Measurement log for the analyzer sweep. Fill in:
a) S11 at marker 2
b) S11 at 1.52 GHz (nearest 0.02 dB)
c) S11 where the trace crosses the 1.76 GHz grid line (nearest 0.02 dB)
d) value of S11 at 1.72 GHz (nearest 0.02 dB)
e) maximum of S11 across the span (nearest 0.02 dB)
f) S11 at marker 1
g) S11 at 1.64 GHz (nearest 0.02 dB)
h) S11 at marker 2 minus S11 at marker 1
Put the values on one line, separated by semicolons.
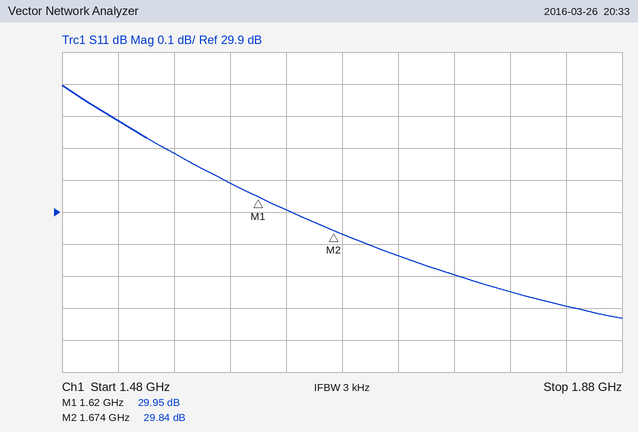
29.84 dB; 30.18 dB; 29.70 dB; 29.76 dB; 30.30 dB; 29.95 dB; 29.90 dB; -0.11 dB
